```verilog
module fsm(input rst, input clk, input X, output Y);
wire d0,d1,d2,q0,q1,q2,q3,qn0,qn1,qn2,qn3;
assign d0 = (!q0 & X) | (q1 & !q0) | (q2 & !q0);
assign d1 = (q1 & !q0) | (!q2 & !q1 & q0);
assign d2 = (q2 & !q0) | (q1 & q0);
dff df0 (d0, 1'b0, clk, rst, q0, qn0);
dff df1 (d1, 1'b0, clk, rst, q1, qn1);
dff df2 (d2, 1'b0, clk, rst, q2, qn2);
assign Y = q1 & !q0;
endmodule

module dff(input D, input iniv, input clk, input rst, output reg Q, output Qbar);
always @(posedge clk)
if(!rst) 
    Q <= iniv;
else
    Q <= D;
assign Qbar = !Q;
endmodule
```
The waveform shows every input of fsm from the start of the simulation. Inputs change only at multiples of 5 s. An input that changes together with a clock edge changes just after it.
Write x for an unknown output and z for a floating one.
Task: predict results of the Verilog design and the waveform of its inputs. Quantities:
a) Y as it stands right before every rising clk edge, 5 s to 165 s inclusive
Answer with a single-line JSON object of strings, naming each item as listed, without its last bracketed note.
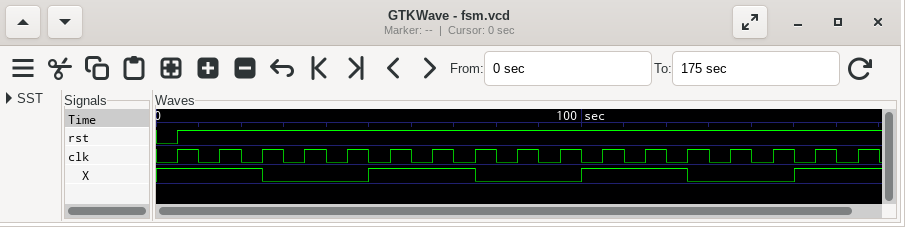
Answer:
{"Y as it stands right before every rising clk edge, 5 s to 165 s inclusive": "x 0 0 1 0 0 0 0 0 1 0 0 0 0 0 0 0"}
